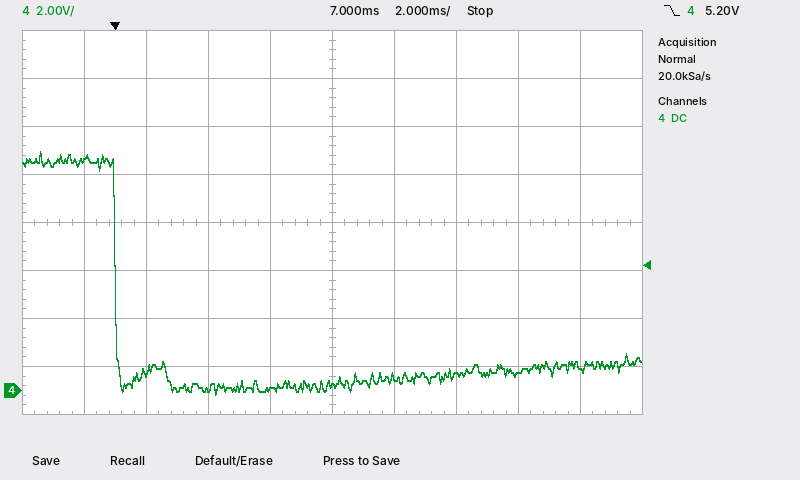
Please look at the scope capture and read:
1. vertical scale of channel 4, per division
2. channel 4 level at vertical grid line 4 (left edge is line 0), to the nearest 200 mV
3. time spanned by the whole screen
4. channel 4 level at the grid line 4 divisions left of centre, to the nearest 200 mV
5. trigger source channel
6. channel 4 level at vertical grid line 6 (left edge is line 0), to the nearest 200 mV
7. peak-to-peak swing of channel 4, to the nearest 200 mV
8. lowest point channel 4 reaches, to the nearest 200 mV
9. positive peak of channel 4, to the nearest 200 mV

2 V
0.0 V
20 ms
9.6 V
channel 4
600 mV
10.2 V
-200 mV
10.0 V
